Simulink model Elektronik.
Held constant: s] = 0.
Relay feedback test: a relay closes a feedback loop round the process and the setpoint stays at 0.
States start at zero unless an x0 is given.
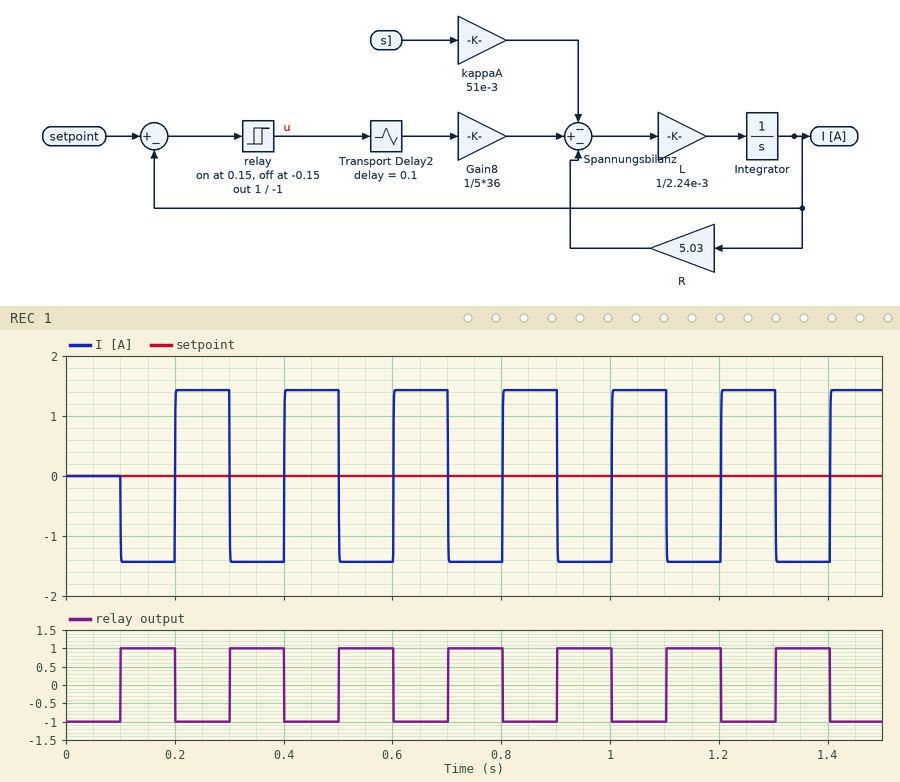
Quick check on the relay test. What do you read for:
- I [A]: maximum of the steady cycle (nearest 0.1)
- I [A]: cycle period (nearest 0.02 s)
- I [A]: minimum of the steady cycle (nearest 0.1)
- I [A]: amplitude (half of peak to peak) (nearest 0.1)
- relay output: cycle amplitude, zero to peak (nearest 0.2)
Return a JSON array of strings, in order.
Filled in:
["1.4", "0.20 s", "-1.4", "1.4", "1.0"]
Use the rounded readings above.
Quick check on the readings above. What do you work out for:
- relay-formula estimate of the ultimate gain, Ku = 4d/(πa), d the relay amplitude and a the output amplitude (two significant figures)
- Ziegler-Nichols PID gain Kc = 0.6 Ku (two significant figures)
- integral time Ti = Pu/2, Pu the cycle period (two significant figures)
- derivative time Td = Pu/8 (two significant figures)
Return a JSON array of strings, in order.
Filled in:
["0.91", "0.55", "0.10 s", "0.025 s"]
